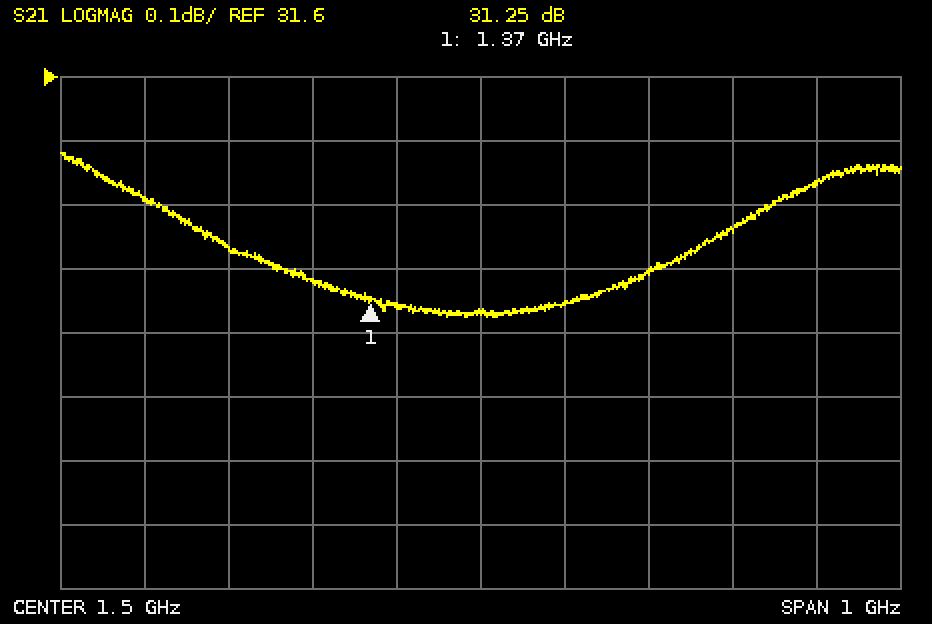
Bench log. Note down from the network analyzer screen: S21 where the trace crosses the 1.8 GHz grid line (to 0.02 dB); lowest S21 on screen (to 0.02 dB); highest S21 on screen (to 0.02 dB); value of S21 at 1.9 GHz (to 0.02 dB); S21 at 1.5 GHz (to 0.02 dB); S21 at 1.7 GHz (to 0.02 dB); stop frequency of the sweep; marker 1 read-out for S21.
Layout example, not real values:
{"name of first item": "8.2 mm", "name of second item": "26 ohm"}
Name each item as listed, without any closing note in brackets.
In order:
{"S21 where the trace crosses the 1.8 GHz grid line": "31.36 dB", "lowest S21 on screen": "31.22 dB", "highest S21 on screen": "31.48 dB", "value of S21 at 1.9 GHz": "31.44 dB", "S21 at 1.5 GHz": "31.24 dB", "S21 at 1.7 GHz": "31.30 dB", "stop frequency of the sweep": "2 GHz", "marker 1 read-out for S21": "31.25 dB"}
